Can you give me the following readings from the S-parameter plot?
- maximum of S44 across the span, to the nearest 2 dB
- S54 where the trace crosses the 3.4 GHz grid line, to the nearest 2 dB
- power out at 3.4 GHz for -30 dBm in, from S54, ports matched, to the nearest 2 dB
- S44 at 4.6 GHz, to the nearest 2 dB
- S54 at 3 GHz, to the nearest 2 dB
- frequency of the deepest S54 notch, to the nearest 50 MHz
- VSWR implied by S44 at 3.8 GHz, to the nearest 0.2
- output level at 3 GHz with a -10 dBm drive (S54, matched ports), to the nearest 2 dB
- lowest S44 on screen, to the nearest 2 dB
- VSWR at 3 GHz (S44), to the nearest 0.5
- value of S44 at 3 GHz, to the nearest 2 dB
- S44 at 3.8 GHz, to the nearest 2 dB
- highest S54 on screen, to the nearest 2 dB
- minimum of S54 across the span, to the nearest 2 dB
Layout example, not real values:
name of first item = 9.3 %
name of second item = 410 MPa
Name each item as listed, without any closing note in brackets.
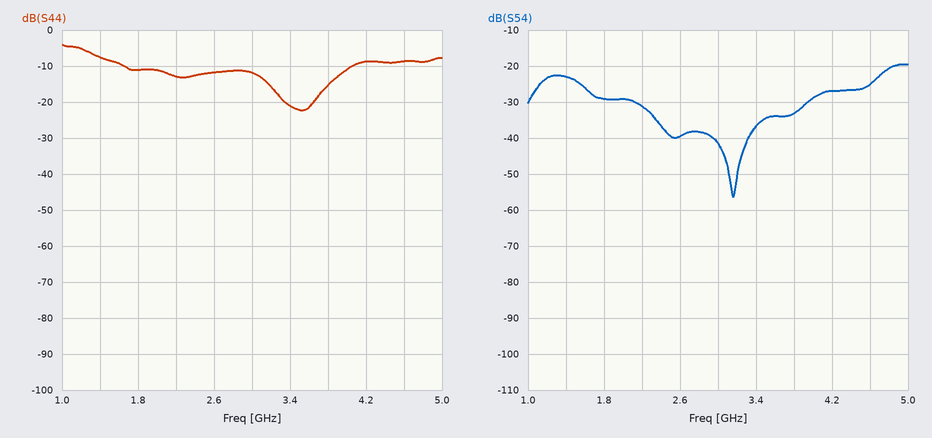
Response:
maximum of S44 across the span, to the nearest 2 dB = -4 dB
S54 where the trace crosses the 3.4 GHz grid line, to the nearest 2 dB = -36 dB
power out at 3.4 GHz for -30 dBm in, from S54, ports matched, to the nearest 2 dB = -66 dBm
S44 at 4.6 GHz, to the nearest 2 dB = -8 dB
S54 at 3 GHz, to the nearest 2 dB = -42 dB
frequency of the deepest S54 notch, to the nearest 50 MHz = 3.15 GHz
VSWR implied by S44 at 3.8 GHz, to the nearest 0.2 = 1.4
output level at 3 GHz with a -10 dBm drive (S54, matched ports), to the nearest 2 dB = -52 dBm
lowest S44 on screen, to the nearest 2 dB = -22 dB
VSWR at 3 GHz (S44), to the nearest 0.5 = 1.5
value of S44 at 3 GHz, to the nearest 2 dB = -12 dB
S44 at 3.8 GHz, to the nearest 2 dB = -16 dB
highest S54 on screen, to the nearest 2 dB = -20 dB
minimum of S54 across the span, to the nearest 2 dB = -56 dB
